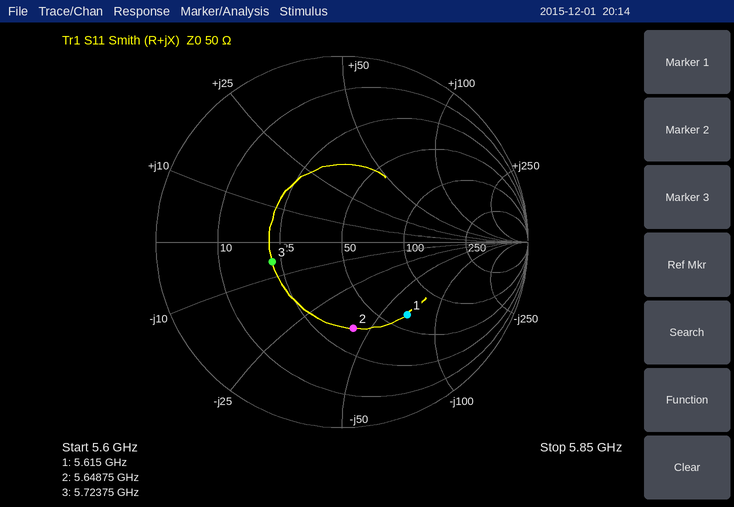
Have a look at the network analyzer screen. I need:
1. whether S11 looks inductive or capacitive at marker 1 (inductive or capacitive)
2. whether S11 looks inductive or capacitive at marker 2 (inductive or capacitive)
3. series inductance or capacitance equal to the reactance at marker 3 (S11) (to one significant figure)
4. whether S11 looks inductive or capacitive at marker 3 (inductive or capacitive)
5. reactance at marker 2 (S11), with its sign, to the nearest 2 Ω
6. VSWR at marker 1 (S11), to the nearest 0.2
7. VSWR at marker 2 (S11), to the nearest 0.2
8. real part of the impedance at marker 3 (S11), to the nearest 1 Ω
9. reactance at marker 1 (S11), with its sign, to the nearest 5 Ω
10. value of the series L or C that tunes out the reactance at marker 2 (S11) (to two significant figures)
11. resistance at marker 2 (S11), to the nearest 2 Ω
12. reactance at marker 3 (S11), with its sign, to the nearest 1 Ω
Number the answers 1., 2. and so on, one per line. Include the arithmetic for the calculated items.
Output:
1. capacitive
2. capacitive
3. C = 1/(2π × 5.72375 GHz × 6 Ω) ≈ 5 pF
4. capacitive
5. -42 Ω
6. 3.2
7. 2.8
8. 22 Ω
9. -70 Ω
10. L = 42 Ω/(2π × 5.64875 GHz) ≈ 1.2 nH
11. 36 Ω
12. -6 Ω
